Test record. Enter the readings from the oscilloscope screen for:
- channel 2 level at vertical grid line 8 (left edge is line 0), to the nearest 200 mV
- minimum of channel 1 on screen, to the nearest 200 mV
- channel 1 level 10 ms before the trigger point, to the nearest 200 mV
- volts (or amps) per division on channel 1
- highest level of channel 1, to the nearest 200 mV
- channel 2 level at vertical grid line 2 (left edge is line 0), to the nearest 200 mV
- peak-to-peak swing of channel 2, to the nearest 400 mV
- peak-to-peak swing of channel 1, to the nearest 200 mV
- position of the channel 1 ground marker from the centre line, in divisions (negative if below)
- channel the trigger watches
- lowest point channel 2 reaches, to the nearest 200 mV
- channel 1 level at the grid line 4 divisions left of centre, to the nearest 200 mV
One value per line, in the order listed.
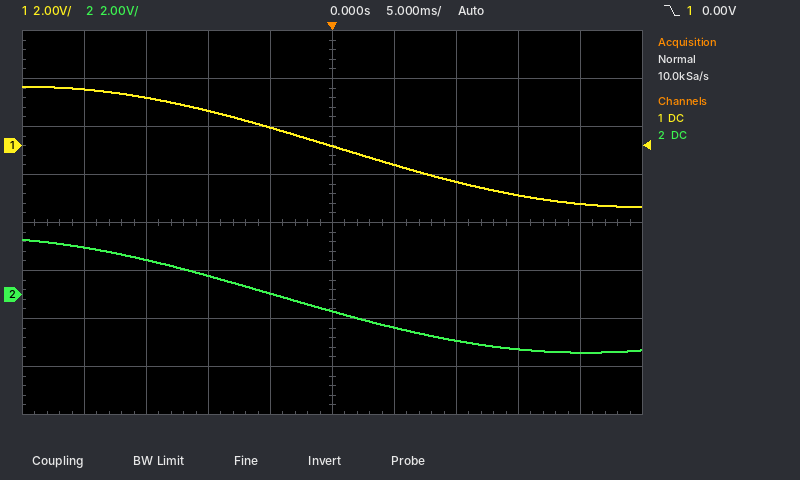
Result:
-2.2 V
-2.6 V
1.4 V
2 V
2.4 V
1.4 V
4.8 V
5.0 V
+1.6 div
channel 1
-2.4 V
2.4 V
